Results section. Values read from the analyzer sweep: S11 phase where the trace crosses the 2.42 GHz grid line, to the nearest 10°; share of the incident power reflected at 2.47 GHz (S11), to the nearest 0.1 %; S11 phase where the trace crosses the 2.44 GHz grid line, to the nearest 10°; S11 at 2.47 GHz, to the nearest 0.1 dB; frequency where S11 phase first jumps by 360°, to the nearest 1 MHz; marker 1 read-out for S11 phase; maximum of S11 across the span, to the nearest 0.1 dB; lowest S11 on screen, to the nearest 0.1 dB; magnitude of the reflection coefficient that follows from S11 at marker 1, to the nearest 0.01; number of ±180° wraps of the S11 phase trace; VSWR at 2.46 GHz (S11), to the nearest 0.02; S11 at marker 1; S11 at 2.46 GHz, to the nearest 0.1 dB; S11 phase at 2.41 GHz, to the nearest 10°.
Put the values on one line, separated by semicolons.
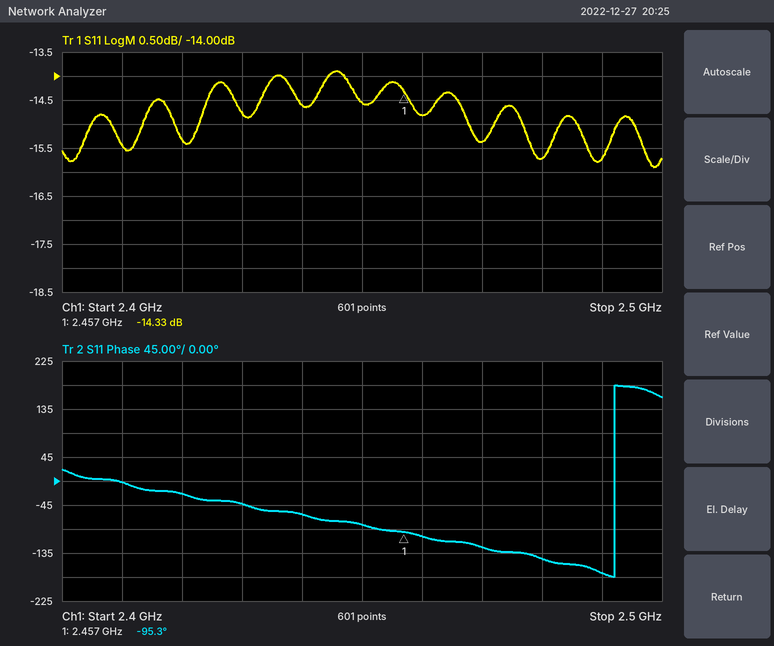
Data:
-20°; 2.9 %; -60°; -15.4 dB; 2.492 GHz; -95.3°; -13.9 dB; -15.9 dB; 0.19; 1; 1.44; -14.33 dB; -14.8 dB; 0°
